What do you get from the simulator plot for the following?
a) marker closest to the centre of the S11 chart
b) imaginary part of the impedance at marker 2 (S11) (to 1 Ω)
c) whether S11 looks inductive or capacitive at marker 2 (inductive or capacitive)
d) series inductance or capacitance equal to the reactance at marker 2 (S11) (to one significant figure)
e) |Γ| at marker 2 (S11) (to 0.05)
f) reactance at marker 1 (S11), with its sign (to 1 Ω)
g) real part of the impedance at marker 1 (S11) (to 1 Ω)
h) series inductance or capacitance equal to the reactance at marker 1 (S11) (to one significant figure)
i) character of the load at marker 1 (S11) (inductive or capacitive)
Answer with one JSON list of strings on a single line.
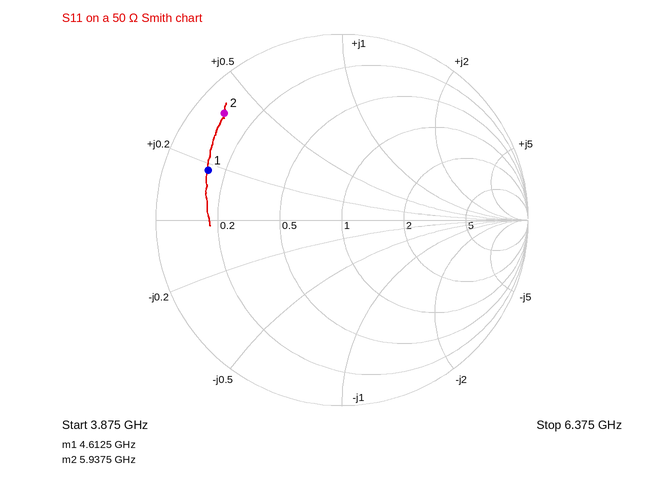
["marker 1", "+19 Ω", "inductive", "500 pH", "0.85", "+9 Ω", "7 Ω", "300 pH", "inductive"]
